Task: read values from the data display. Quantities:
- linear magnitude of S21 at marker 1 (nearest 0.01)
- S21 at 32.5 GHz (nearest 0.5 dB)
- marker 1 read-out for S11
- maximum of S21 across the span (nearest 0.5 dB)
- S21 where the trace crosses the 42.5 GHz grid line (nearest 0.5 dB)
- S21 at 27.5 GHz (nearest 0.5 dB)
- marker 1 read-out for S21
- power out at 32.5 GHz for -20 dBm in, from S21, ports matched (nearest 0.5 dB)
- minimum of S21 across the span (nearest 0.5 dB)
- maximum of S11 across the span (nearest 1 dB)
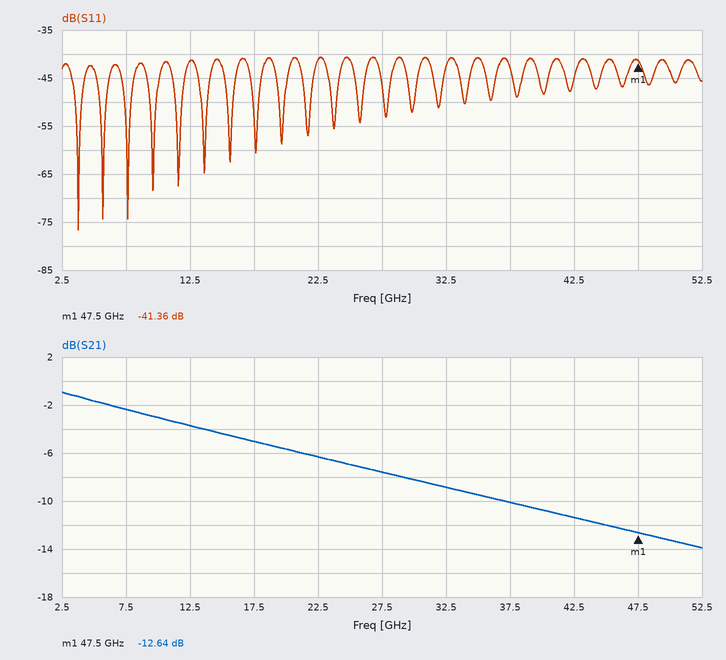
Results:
0.23
-9.0 dB
-41.36 dB
-1.0 dB
-11.5 dB
-7.5 dB
-12.64 dB
-29.0 dBm
-14.0 dB
-41 dB
